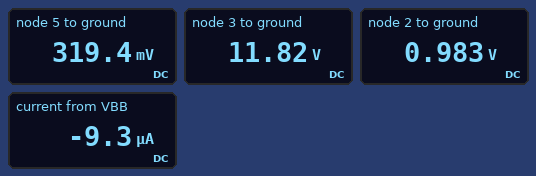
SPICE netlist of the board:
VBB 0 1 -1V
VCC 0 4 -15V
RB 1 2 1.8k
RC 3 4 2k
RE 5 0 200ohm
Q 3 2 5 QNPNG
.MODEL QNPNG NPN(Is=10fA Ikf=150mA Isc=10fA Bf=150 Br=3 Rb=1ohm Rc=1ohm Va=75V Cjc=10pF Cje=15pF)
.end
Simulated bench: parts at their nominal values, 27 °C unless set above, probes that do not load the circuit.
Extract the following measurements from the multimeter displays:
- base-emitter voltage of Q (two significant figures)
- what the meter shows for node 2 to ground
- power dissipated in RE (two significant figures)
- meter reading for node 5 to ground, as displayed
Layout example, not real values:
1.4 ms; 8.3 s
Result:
660 mV; 0.983 V; 510 µW; 319.4 mV
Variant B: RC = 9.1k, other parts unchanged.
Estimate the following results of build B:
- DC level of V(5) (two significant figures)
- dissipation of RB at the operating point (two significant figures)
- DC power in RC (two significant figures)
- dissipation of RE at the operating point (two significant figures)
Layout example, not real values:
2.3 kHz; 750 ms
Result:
310 mV; 200 nW; 22 mW; 490 µW
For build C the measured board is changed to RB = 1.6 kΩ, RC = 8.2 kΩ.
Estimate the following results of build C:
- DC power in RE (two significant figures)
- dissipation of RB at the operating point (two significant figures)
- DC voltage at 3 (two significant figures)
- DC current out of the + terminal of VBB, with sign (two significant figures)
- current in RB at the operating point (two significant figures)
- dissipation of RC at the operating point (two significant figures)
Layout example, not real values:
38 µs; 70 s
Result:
500 µW; 170 nW; 2.1 V; -10 µA; 10 µA; 20 mW
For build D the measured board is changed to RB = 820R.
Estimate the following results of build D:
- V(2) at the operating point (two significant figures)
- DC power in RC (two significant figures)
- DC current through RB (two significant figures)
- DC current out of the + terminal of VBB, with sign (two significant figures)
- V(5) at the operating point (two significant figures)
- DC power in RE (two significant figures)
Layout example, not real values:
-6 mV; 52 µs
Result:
990 mV; 5.3 mW; 9.6 µA; -9.6 µA; 330 mV; 540 µW
